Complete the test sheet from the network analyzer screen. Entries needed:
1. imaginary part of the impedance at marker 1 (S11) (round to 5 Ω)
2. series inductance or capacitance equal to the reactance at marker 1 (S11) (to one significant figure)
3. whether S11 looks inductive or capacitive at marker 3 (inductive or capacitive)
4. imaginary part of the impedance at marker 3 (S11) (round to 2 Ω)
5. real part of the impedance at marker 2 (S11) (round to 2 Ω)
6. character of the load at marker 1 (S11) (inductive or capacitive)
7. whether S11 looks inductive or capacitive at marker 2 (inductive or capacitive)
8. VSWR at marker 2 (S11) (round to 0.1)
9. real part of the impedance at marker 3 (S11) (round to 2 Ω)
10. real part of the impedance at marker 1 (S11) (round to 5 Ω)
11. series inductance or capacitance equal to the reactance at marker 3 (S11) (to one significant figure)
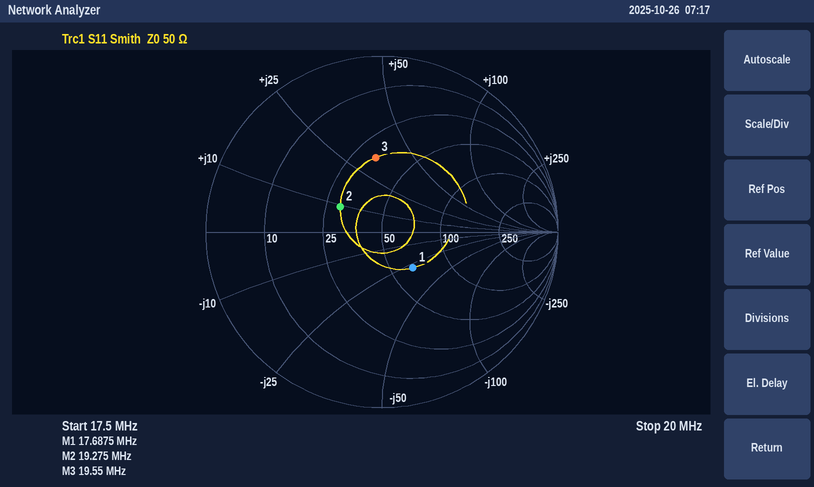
-30 Ω
300 pF
inductive
+34 Ω
30 Ω
capacitive
inductive
1.8
32 Ω
65 Ω
300 nH
